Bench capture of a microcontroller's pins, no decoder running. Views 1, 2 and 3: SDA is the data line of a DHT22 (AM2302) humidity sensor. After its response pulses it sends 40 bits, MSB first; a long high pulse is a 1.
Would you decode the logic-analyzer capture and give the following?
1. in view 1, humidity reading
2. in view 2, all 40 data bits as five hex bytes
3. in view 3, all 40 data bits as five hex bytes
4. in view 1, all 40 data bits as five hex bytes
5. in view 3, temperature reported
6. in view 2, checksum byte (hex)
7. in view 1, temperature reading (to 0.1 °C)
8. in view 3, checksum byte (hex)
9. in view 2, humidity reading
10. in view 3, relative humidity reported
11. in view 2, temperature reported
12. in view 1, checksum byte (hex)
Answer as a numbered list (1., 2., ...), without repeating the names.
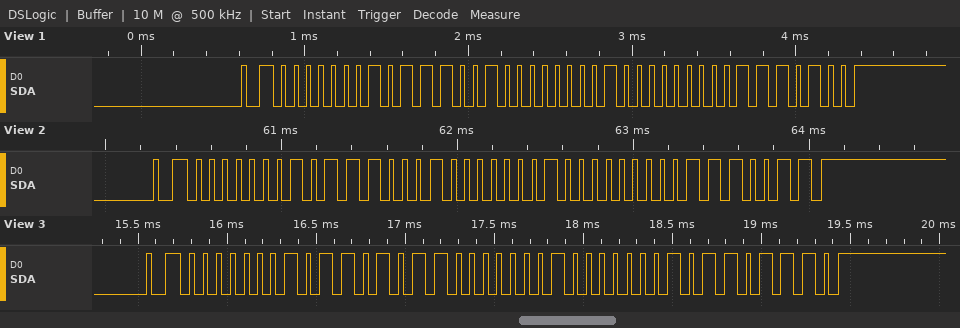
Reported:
1. 37.0 %
2. 01 71 01 00 73
3. 01 6B 01 01 6E
4. 01 72 01 00 74
5. 25.7 °C
6. 0x73
7. 25.6 °C
8. 0x6E
9. 36.9 %
10. 36.3 %
11. 25.6 °C
12. 0x74
